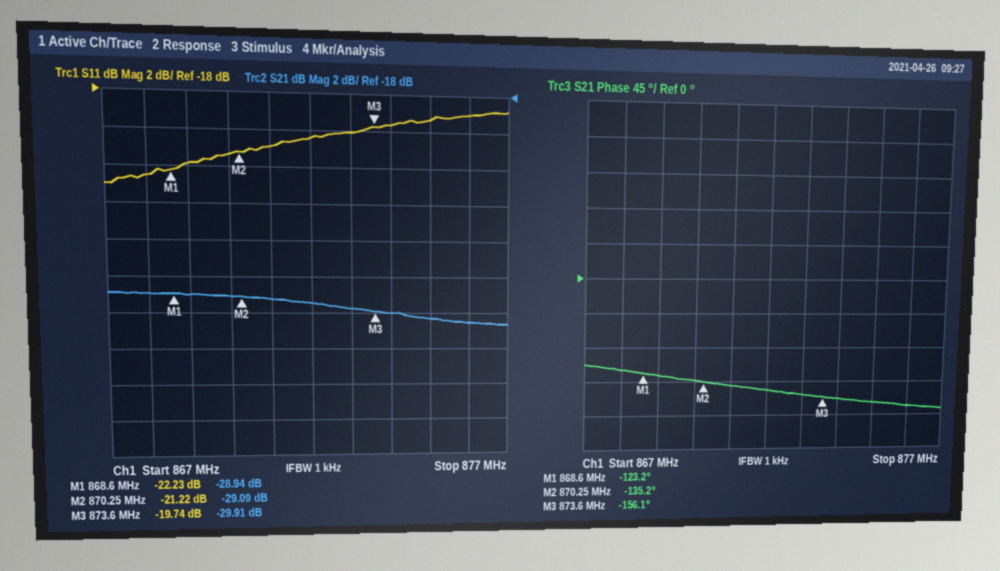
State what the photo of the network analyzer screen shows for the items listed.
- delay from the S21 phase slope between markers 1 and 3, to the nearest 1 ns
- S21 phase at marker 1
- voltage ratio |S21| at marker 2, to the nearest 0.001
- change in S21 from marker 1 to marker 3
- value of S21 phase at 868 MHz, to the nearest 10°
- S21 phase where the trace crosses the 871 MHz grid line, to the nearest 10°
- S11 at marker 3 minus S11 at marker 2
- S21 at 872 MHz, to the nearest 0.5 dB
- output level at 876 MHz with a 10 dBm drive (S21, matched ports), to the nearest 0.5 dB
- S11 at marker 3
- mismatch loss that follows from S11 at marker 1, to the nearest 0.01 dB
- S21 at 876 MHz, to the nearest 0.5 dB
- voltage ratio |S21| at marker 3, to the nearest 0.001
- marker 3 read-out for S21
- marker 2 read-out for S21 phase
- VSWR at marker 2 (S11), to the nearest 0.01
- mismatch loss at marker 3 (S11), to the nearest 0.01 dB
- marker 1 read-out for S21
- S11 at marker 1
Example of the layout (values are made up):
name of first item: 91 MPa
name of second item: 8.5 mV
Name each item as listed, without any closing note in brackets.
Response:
delay from the S21 phase slope between markers 1 and 3, to the nearest 1 ns: 18 ns
S21 phase at marker 1: -123.2°
voltage ratio |S21| at marker 2, to the nearest 0.001: 0.035
change in S21 from marker 1 to marker 3: -0.97 dB
value of S21 phase at 868 MHz, to the nearest 10°: -120°
S21 phase where the trace crosses the 871 MHz grid line, to the nearest 10°: -140°
S11 at marker 3 minus S11 at marker 2: 1.48 dB
S21 at 872 MHz, to the nearest 0.5 dB: -29.5 dB
output level at 876 MHz with a 10 dBm drive (S21, matched ports), to the nearest 0.5 dB: -20.5 dBm
S11 at marker 3: -19.74 dB
mismatch loss that follows from S11 at marker 1, to the nearest 0.01 dB: 0.03 dB
S21 at 876 MHz, to the nearest 0.5 dB: -30.5 dB
voltage ratio |S21| at marker 3, to the nearest 0.001: 0.032
marker 3 read-out for S21: -29.91 dB
marker 2 read-out for S21 phase: -135.2°
VSWR at marker 2 (S11), to the nearest 0.01: 1.19
mismatch loss at marker 3 (S11), to the nearest 0.01 dB: 0.05 dB
marker 1 read-out for S21: -28.94 dB
S11 at marker 1: -22.23 dB
